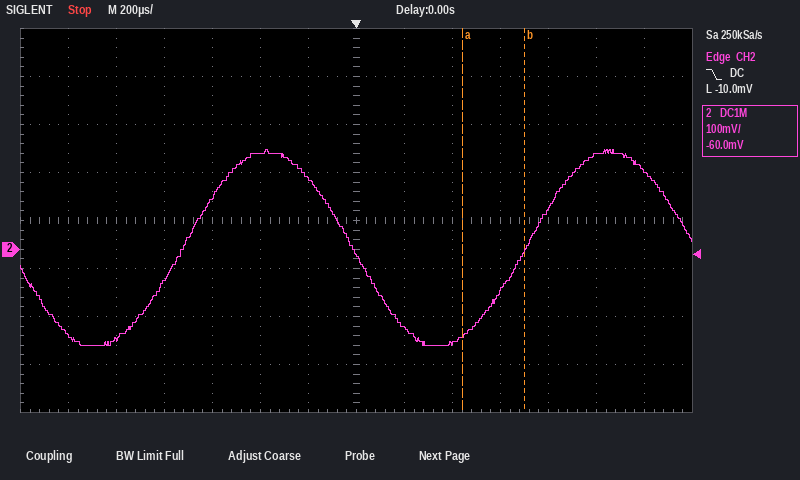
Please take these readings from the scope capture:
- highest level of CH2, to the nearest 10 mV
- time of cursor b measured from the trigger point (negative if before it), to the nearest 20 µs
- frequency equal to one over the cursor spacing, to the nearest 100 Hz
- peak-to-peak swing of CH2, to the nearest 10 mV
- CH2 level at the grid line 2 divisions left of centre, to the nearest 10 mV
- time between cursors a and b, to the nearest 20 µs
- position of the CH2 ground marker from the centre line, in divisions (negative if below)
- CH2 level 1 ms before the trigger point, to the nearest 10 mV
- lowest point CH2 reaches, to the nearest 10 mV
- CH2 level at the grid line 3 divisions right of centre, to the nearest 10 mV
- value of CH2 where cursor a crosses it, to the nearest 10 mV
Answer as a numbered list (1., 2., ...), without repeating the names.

1. 210 mV
2. +700 µs
3. 3.8 kHz
4. 410 mV
5. 200 mV
6. 260 µs
7. -0.6 div
8. -190 mV
9. -200 mV
10. -90 mV
11. -180 mV
